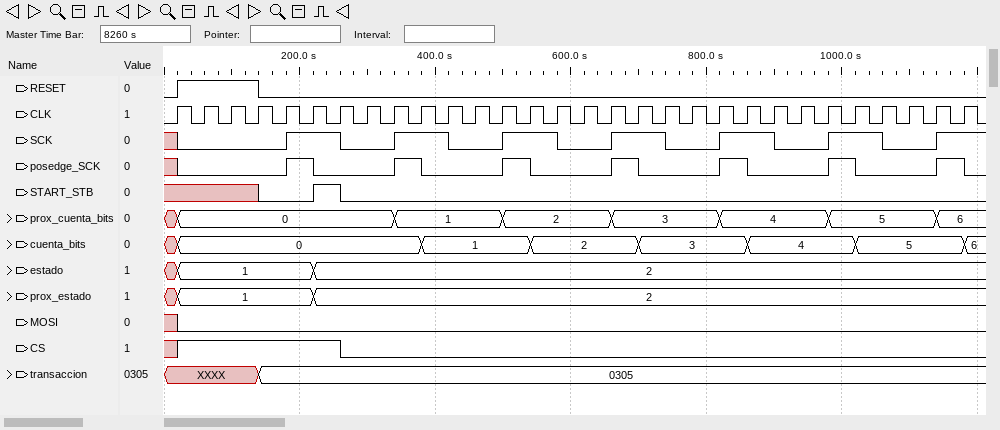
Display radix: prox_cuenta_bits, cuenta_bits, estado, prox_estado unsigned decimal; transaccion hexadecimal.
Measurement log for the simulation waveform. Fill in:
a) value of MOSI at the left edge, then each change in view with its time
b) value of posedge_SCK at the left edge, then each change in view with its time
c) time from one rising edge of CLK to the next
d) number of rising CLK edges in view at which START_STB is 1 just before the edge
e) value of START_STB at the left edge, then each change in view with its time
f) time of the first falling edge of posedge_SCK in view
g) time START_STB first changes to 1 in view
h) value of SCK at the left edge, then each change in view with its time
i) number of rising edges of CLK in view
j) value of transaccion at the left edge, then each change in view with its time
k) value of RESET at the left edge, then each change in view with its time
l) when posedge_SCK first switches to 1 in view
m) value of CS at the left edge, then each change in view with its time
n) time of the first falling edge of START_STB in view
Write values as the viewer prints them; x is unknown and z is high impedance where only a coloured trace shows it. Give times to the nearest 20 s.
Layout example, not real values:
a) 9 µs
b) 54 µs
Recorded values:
a) x, 0 at 20 s
b) x, 0 at 20 s, 1 at 180 s, 0 at 220 s, 1 at 340 s, 0 at 380 s, 1 at 500 s, 0 at 540 s, 1 at 660 s, 0 at 700 s, 1 at 820 s, 0 at 860 s, 1 at 980 s, 0 at 1020 s, 1 at 1140 s, 0 at 1180 s
c) 40 s
d) 1
e) x, 0 at 140 s, 1 at 220 s, 0 at 260 s
f) 220 s
g) 220 s
h) x, 0 at 20 s, 1 at 180 s, 0 at 260 s, 1 at 340 s, 0 at 420 s, 1 at 500 s, 0 at 580 s, 1 at 660 s, 0 at 740 s, 1 at 820 s, 0 at 900 s, 1 at 980 s, 0 at 1060 s, 1 at 1140 s
i) 30
j) XXXX, 0305 at 140 s
k) 0, 1 at 20 s, 0 at 140 s
l) 180 s
m) x, 1 at 20 s, 0 at 260 s
n) 260 s
